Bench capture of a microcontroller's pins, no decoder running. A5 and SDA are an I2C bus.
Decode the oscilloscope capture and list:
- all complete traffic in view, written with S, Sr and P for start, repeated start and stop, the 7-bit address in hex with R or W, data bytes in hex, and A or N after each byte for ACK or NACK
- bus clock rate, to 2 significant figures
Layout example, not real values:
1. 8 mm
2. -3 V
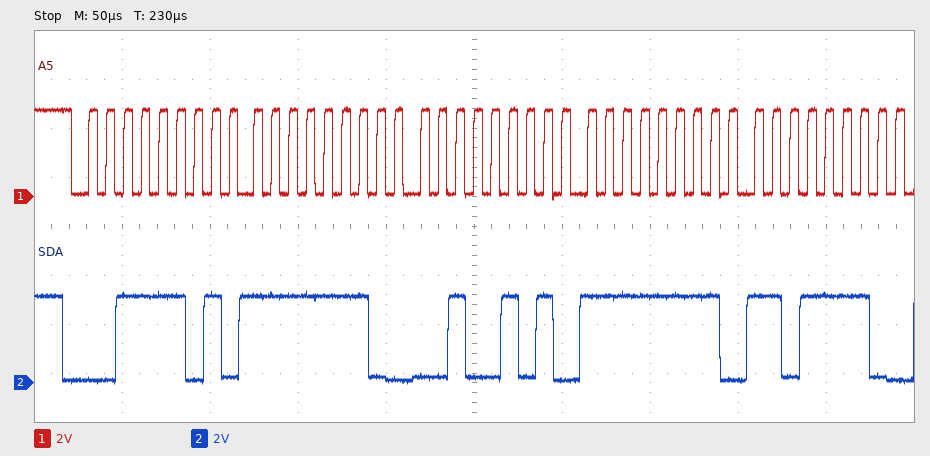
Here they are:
1. S 1ER A FE A 25 A FF A DE A
2. 100 kHz
